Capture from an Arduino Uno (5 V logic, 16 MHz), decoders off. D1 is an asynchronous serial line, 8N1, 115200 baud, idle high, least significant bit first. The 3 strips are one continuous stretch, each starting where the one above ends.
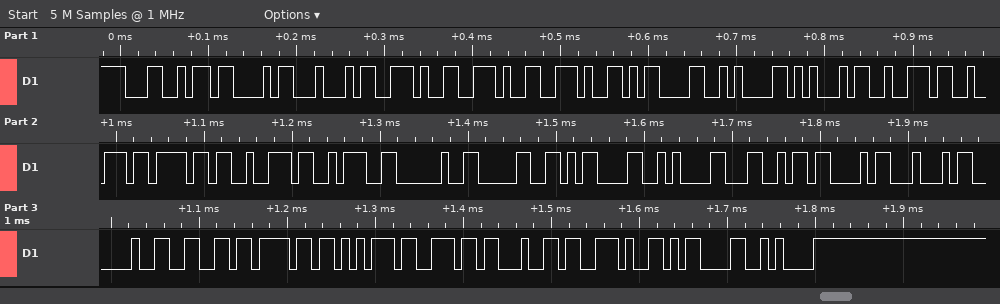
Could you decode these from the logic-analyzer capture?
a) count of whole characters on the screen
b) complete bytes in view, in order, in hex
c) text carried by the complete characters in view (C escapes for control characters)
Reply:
30
4C 43 44 2E 2E 2E 0D 0A 45 72 72 6F 72 3A 20 30 0D 0A 4C 43 44 20 66 6F 75 6E 64 2E 0D 0A
"LCD...\r\nError: 0\r\nLCD found.\r\n"
